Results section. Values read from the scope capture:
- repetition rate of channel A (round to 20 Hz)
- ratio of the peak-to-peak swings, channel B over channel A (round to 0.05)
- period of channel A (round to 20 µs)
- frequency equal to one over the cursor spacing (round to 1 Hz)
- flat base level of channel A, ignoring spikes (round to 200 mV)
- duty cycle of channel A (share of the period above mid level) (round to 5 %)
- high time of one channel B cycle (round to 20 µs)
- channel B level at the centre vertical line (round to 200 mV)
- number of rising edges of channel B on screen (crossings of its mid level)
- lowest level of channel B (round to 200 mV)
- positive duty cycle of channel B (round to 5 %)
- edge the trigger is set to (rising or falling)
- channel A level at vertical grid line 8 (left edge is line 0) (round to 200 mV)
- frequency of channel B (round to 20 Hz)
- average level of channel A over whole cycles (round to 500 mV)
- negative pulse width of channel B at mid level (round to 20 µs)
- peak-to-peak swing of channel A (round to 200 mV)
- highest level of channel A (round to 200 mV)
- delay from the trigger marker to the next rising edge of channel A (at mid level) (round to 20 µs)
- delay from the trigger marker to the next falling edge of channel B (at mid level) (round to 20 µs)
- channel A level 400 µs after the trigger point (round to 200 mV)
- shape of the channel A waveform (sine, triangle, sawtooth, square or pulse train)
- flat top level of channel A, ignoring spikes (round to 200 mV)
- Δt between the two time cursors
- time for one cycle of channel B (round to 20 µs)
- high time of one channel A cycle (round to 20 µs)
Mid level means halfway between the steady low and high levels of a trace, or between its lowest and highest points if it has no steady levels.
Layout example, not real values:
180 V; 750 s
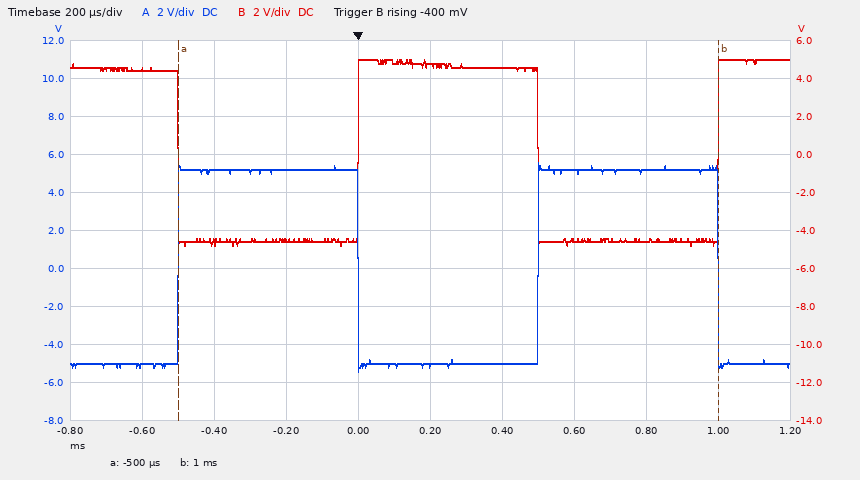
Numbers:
1.00 kHz; 0.90; 1.00 ms; 667 Hz; -5.0 V; 50 %; 500 µs; 4.8 V; 2; -4.8 V; 50 %; rising; 5.2 V; 1.00 kHz; 0.0 V; 500 µs; 11.0 V; 5.6 V; 500 µs; 500 µs; -5.0 V; square; 5.2 V; 1.50 ms; 1.00 ms; 500 µs
